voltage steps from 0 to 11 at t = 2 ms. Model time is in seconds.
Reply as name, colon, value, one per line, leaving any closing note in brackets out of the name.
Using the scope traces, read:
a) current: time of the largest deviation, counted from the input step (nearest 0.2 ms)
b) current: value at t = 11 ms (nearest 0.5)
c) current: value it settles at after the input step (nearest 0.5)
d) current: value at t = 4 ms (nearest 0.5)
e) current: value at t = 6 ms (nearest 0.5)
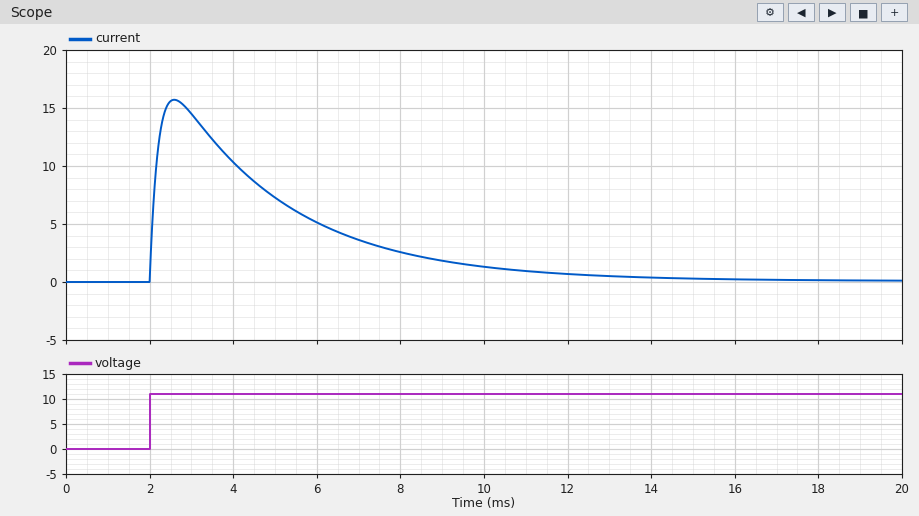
current: time of the largest deviation, counted from the input step: 0.6 ms
current: value at t = 11 ms: 1.0
current: value it settles at after the input step: 0.0
current: value at t = 4 ms: 10.5
current: value at t = 6 ms: 5.0
